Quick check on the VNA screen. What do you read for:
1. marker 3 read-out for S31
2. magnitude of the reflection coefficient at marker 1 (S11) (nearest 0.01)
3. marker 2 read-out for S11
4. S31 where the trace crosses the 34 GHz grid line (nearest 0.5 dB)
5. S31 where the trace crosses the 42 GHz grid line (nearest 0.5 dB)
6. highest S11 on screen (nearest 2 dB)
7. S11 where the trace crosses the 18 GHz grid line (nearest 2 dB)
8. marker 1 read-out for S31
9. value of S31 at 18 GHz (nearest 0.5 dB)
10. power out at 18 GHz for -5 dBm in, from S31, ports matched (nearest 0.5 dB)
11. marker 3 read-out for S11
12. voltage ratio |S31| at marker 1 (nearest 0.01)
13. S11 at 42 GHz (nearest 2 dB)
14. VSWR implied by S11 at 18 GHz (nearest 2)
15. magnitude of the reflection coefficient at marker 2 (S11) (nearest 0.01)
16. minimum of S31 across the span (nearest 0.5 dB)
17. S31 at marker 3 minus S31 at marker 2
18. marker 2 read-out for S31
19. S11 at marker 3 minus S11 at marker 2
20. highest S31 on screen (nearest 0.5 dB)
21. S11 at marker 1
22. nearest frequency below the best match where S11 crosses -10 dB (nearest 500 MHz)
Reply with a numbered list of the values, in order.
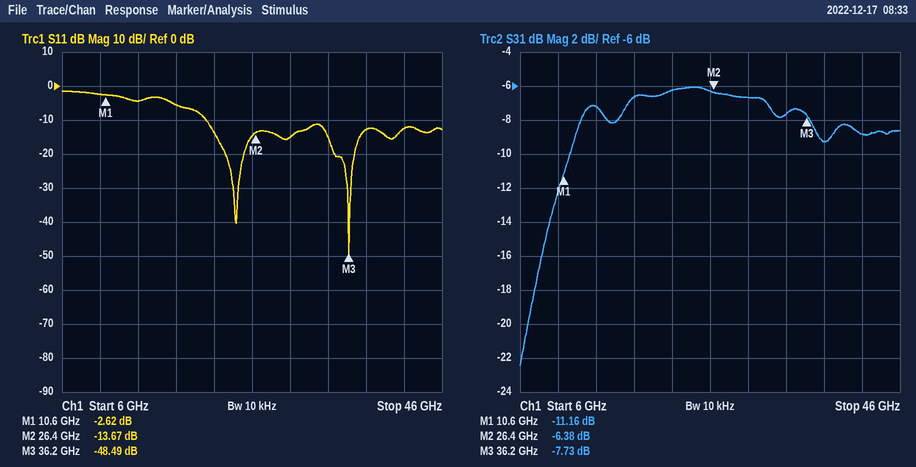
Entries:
1. -7.73 dB
2. 0.74
3. -13.67 dB
4. -7.5 dB
5. -9.0 dB
6. -2 dB
7. -6 dB
8. -11.16 dB
9. -6.5 dB
10. -11.5 dBm
11. -48.49 dB
12. 0.28
13. -12 dB
14. 4
15. 0.21
16. -22.5 dB
17. -1.35 dB
18. -6.38 dB
19. -34.82 dB
20. -6.0 dB
21. -2.62 dB
22. 21.0 GHz
